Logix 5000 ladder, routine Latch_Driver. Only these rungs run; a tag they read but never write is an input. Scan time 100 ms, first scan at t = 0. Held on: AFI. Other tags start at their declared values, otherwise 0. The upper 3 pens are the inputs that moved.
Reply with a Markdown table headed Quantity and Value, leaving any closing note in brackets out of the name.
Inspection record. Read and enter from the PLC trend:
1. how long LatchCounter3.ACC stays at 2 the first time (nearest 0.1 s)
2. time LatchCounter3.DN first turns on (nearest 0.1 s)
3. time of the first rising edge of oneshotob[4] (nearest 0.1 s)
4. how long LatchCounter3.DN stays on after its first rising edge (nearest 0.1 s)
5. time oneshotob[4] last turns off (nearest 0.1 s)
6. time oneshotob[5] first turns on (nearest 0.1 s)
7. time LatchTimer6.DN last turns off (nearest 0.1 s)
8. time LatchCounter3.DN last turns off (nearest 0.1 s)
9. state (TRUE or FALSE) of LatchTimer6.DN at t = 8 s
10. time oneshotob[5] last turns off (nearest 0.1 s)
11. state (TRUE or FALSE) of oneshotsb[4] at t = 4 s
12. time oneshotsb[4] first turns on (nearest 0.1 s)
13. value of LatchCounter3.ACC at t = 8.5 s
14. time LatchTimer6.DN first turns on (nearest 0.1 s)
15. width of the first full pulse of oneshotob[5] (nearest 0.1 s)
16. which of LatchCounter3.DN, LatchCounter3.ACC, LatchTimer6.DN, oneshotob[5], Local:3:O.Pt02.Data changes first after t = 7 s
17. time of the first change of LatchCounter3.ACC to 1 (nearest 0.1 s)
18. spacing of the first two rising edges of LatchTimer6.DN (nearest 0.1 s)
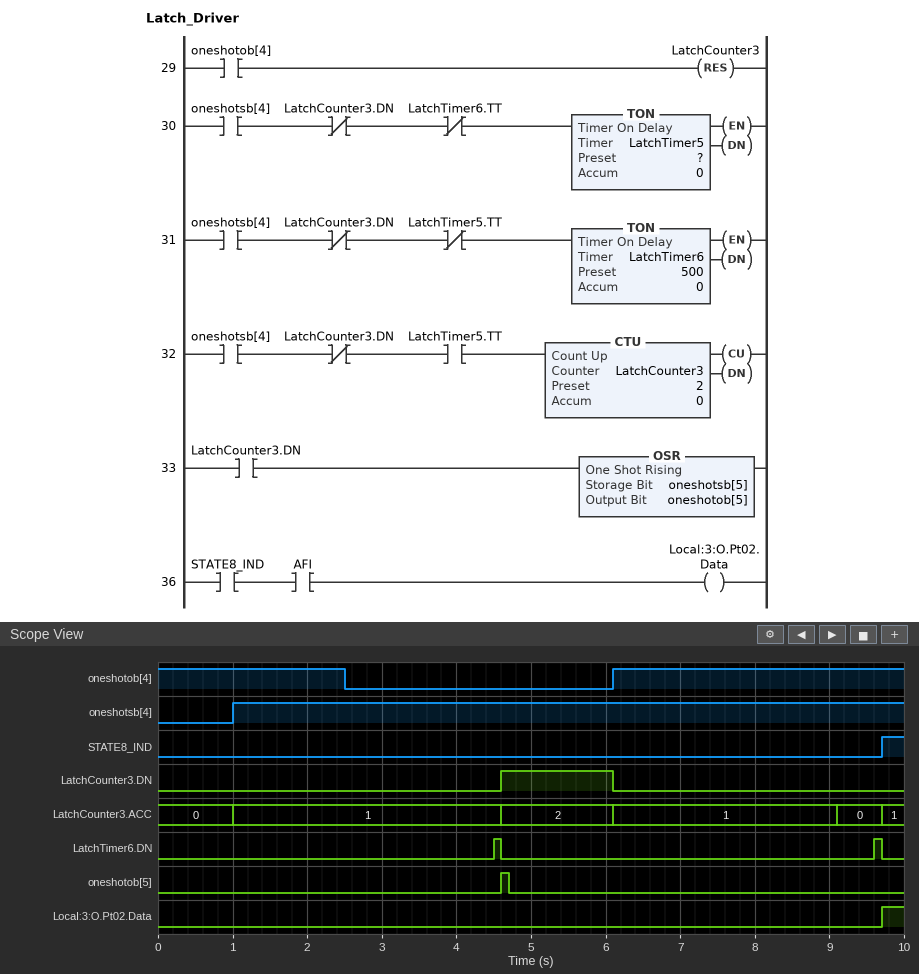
| Quantity | Value |
|---|---|
| how long LatchCounter3.ACC stays at 2 the first time | 1.5 s |
| time LatchCounter3.DN first turns on | 4.6 s |
| time of the first rising edge of oneshotob[4] | 6.1 s |
| how long LatchCounter3.DN stays on after its first rising edge | 1.5 s |
| time oneshotob[4] last turns off | 2.5 s |
| time oneshotob[5] first turns on | 4.6 s |
| time LatchTimer6.DN last turns off | 9.7 s |
| time LatchCounter3.DN last turns off | 6.1 s |
| state (TRUE or FALSE) of LatchTimer6.DN at t = 8 s | FALSE |
| time oneshotob[5] last turns off | 4.7 s |
| state (TRUE or FALSE) of oneshotsb[4] at t = 4 s | TRUE |
| time oneshotsb[4] first turns on | 1.0 s |
| value of LatchCounter3.ACC at t = 8.5 s | 1 |
| time LatchTimer6.DN first turns on | 4.5 s |
| width of the first full pulse of oneshotob[5] | 0.1 s |
| which of LatchCounter3.DN, LatchCounter3.ACC, LatchTimer6.DN, oneshotob[5], Local:3:O.Pt02.Data changes first after t = 7 s | LatchCounter3.ACC |
| time of the first change of LatchCounter3.ACC to 1 | 1.0 s |
| spacing of the first two rising edges of LatchTimer6.DN | 5.1 s |
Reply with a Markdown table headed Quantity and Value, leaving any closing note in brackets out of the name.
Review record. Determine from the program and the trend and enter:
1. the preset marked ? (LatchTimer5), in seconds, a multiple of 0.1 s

| Quantity | Value |
|---|---|
| the preset marked ? (LatchTimer5), in seconds, a multiple of 0.1 s | 3.0 s |
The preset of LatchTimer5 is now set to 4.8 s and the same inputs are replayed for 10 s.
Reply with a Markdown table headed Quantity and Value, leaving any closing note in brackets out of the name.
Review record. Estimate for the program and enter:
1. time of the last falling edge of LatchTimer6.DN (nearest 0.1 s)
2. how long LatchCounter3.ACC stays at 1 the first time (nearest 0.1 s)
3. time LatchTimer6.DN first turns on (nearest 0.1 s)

| Quantity | Value |
|---|---|
| time of the last falling edge of LatchTimer6.DN | 6.4 s |
| how long LatchCounter3.ACC stays at 1 the first time | 5.1 s |
| time LatchTimer6.DN first turns on | 6.3 s |
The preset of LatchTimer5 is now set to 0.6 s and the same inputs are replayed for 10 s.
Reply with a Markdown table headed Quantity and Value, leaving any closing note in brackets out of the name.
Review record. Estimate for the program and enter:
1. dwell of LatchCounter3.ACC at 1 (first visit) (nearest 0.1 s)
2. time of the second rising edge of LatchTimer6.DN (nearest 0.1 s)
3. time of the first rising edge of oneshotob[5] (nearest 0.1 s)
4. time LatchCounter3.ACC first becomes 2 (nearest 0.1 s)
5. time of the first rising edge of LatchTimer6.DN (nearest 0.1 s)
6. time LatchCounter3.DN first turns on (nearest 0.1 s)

| Quantity | Value |
|---|---|
| dwell of LatchCounter3.ACC at 1 (first visit) | 0.6 s |
| time of the second rising edge of LatchTimer6.DN | 3.3 s |
| time of the first rising edge of oneshotob[5] | 3.4 s |
| time LatchCounter3.ACC first becomes 2 | 3.4 s |
| time of the first rising edge of LatchTimer6.DN | 2.1 s |
| time LatchCounter3.DN first turns on | 3.4 s |
